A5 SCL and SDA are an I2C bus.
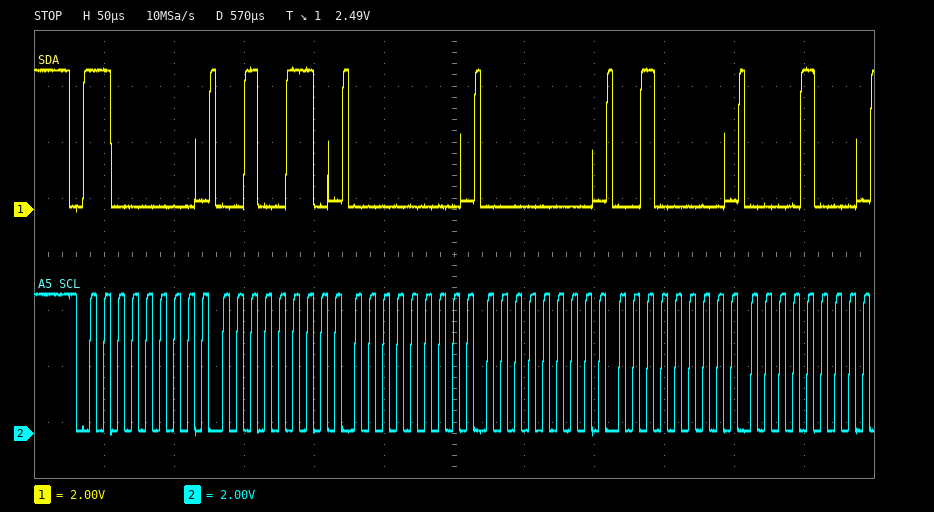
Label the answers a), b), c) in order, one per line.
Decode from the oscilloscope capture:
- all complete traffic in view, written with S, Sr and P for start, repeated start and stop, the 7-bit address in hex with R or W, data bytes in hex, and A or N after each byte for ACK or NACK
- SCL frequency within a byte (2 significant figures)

a) S 60W A 26 A 00 A 00 A 20 A 08 A
b) 100 kHz
